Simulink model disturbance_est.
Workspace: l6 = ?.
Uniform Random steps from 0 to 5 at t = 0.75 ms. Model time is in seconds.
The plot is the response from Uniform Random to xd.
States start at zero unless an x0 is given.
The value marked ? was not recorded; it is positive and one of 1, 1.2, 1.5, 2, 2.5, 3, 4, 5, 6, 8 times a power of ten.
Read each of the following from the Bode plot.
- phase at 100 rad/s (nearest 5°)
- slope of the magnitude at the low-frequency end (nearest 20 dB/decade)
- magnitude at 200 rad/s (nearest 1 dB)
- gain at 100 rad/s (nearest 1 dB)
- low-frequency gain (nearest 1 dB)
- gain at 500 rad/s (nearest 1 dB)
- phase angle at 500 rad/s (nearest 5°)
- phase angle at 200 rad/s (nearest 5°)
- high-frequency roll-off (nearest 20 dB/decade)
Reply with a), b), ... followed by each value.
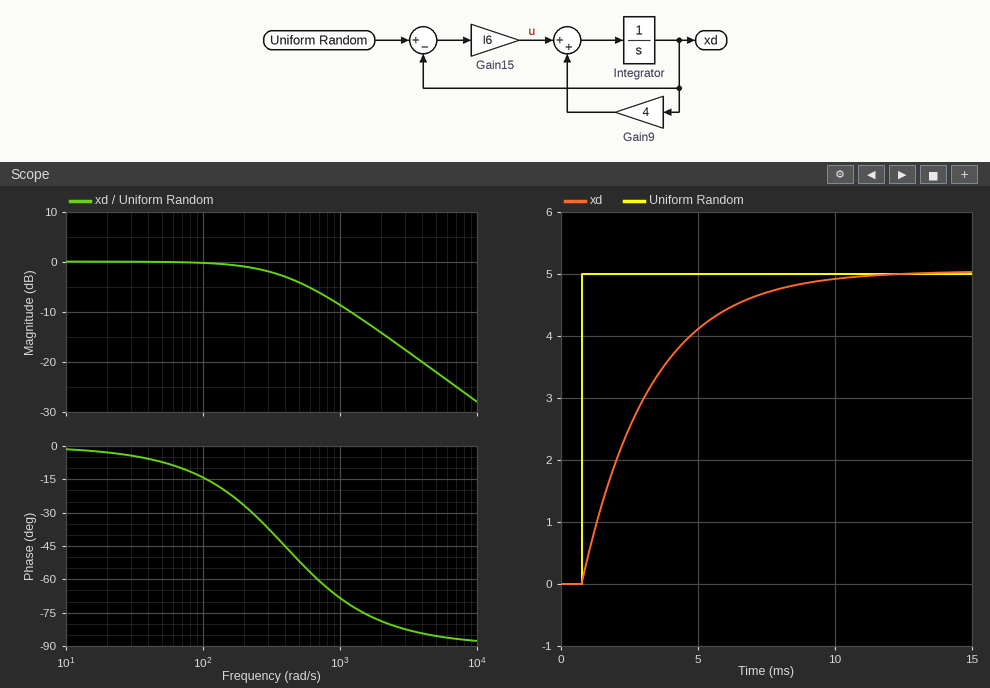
a) -15°
b) 0 dB/decade
c) -1 dB
d) 0 dB
e) 0 dB
f) -4 dB
g) -50°
h) -25°
i) -20 dB/decade
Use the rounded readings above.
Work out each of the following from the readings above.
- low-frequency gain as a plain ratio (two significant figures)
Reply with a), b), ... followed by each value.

a) 1.0
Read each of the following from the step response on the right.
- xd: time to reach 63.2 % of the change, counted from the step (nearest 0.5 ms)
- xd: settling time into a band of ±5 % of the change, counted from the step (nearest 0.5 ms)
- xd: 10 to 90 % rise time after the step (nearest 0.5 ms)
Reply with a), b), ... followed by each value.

a) 2.5 ms
b) 7.5 ms
c) 5.5 ms
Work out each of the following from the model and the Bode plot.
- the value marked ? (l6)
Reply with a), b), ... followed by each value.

a) 400
